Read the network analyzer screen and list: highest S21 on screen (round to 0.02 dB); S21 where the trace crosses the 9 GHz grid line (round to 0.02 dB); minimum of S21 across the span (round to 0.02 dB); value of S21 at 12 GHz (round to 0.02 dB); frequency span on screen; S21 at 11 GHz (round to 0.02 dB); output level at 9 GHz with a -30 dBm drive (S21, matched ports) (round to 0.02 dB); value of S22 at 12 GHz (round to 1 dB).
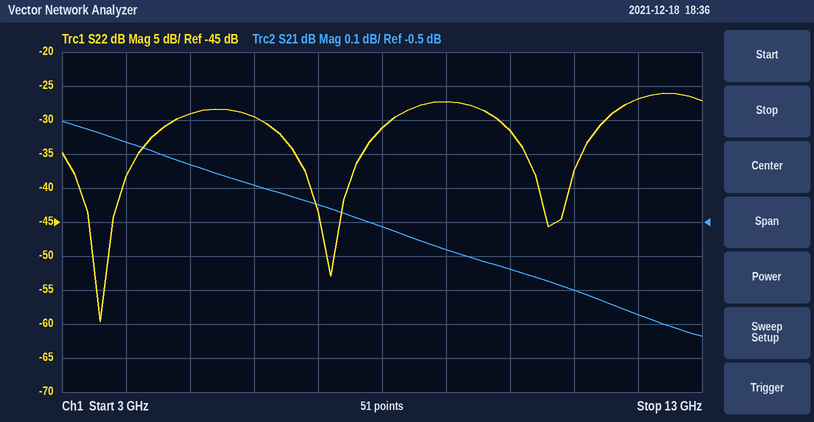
-0.20 dB
-0.58 dB
-0.84 dB
-0.78 dB
10 GHz
-0.70 dB
-30.58 dBm
-27 dB
